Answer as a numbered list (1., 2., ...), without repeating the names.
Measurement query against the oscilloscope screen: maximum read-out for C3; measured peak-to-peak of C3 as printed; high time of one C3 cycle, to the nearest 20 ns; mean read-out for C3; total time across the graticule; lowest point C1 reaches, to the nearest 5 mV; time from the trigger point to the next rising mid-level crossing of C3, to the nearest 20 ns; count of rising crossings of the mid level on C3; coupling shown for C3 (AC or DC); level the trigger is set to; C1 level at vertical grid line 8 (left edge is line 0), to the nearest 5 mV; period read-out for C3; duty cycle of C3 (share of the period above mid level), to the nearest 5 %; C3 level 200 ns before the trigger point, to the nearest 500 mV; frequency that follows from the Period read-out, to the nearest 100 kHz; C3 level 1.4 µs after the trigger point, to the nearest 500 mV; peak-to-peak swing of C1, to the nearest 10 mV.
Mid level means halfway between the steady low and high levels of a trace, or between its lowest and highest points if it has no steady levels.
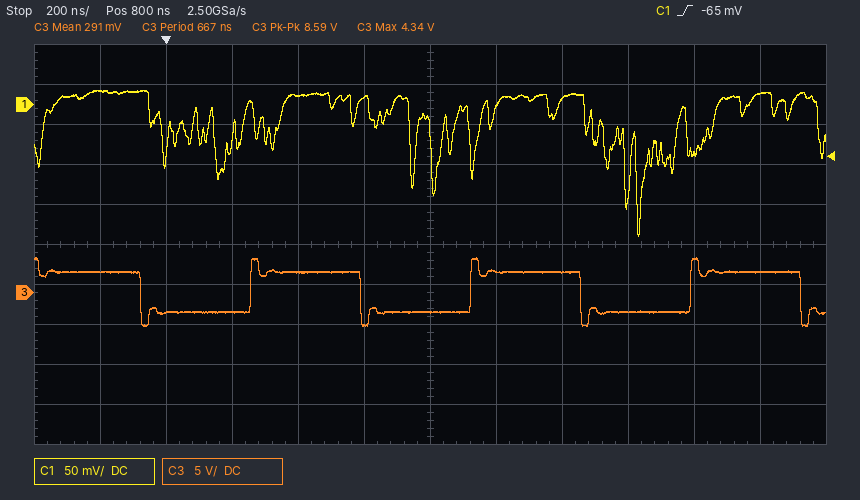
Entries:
1. 4.34 V
2. 8.59 V
3. 340 ns
4. 291 mV
5. 2.4 µs
6. -165 mV
7. 260 ns
8. 3
9. DC
10. -65 mV
11. 5 mV
12. 667 ns
13. 50 %
14. 2.5 V
15. 1.5 MHz
16. -2.5 V
17. 180 mV
